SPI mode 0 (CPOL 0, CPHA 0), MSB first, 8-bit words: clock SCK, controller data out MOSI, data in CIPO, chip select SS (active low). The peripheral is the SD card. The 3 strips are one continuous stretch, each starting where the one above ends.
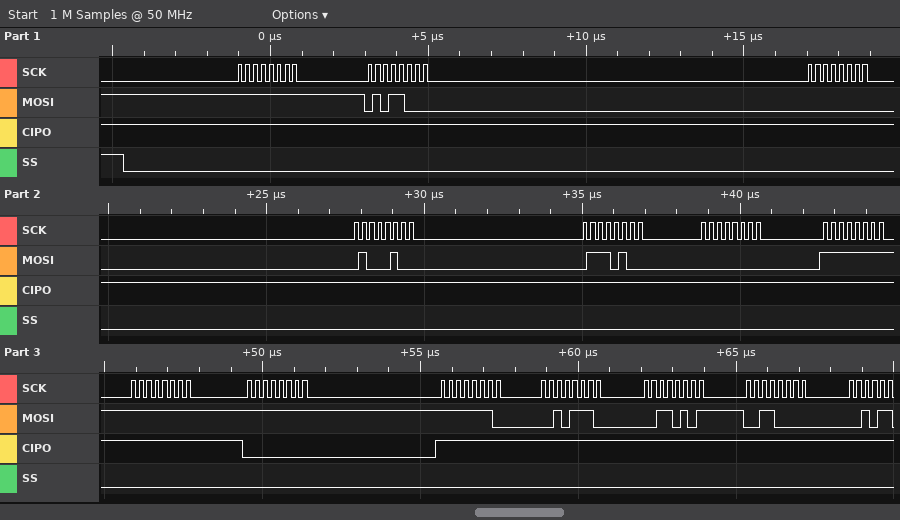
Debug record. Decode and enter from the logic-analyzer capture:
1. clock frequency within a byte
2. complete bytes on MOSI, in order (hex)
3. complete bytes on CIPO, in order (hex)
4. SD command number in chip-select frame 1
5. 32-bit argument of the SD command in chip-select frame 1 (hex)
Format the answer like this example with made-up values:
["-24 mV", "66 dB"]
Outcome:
["4 MHz", "0xFF 0x58 0x00 0x44 0x74 0x00 0xFF 0xFF 0xFF 0xFE 0x2E 0x35 0x30", "0xFF 0xFF 0xFF 0xFF 0xFF 0xFF 0xFF 0xFF 0x00 0xFF 0xFF 0xFF 0xFF", "CMD24", "0x00447400"]
